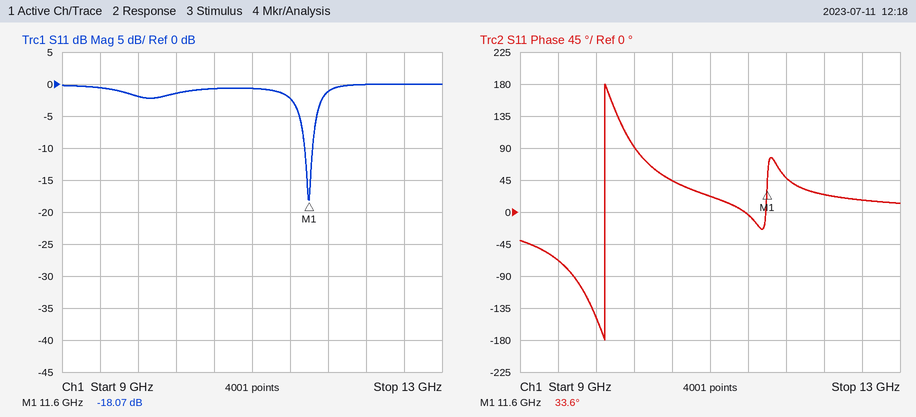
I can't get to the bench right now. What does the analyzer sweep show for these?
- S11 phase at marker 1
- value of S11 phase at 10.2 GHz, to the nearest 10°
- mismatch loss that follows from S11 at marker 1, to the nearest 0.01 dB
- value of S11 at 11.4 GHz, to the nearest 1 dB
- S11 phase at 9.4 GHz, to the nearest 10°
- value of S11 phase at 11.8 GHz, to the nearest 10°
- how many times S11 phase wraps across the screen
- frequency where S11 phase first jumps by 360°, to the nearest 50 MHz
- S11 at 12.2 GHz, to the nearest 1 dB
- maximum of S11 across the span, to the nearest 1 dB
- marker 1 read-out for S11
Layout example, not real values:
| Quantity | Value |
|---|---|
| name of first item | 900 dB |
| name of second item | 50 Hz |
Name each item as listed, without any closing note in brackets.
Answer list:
| Quantity | Value |
|---|---|
| S11 phase at marker 1 | 33.6° |
| value of S11 phase at 10.2 GHz, to the nearest 10° | 90° |
| mismatch loss that follows from S11 at marker 1, to the nearest 0.01 dB | 0.07 dB |
| value of S11 at 11.4 GHz, to the nearest 1 dB | -2 dB |
| S11 phase at 9.4 GHz, to the nearest 10° | -70° |
| value of S11 phase at 11.8 GHz, to the nearest 10° | 50° |
| how many times S11 phase wraps across the screen | 1 |
| frequency where S11 phase first jumps by 360°, to the nearest 50 MHz | 9.90 GHz |
| S11 at 12.2 GHz, to the nearest 1 dB | 0 dB |
| maximum of S11 across the span, to the nearest 1 dB | 0 dB |
| marker 1 read-out for S11 | -18.07 dB |
